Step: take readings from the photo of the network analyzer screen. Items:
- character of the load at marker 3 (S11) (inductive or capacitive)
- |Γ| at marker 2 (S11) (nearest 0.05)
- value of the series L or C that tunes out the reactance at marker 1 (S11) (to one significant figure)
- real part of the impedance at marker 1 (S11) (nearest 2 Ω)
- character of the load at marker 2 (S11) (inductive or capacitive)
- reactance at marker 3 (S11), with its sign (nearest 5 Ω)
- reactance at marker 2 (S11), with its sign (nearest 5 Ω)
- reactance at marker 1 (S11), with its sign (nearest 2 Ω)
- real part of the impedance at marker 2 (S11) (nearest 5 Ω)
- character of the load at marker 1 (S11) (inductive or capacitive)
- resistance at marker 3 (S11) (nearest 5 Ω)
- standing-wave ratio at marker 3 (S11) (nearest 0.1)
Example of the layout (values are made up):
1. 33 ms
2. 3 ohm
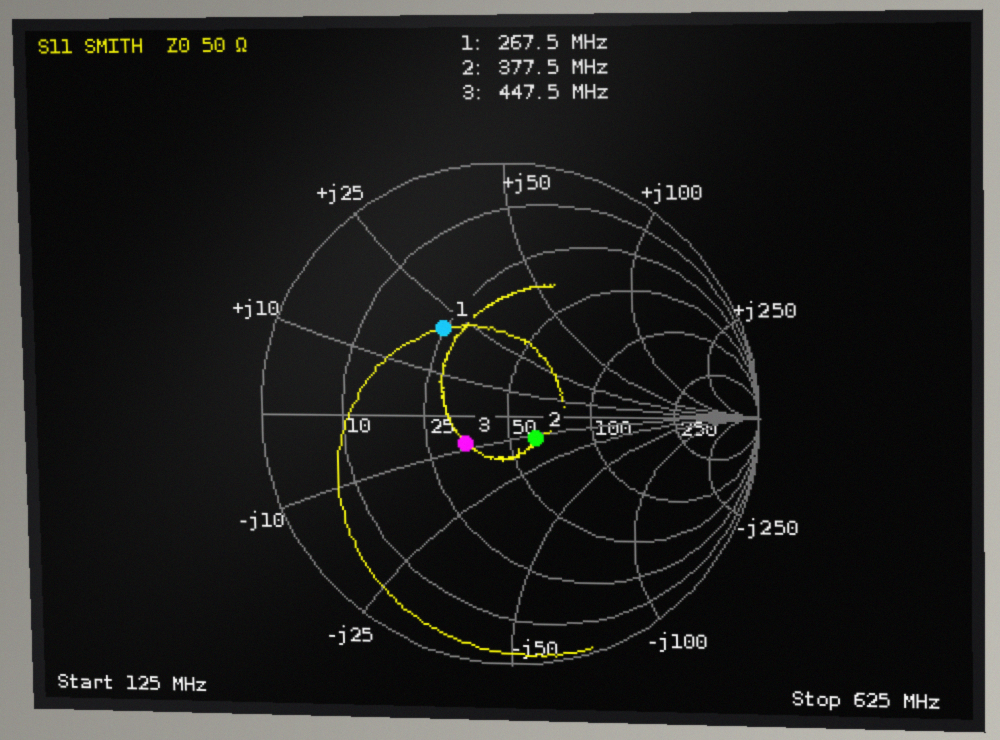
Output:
1. capacitive
2. 0.15
3. 30 pF
4. 24 Ω
5. capacitive
6. -10 Ω
7. -10 Ω
8. +20 Ω
9. 60 Ω
10. inductive
11. 35 Ω
12. 1.5
